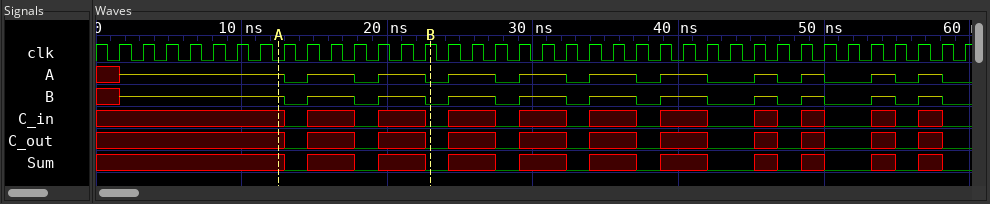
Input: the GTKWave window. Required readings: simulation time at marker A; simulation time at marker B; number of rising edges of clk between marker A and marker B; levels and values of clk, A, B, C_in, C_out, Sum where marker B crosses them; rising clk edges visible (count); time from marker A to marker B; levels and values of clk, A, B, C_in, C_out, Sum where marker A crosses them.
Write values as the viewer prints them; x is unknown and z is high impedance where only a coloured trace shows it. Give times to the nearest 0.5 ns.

12.5 ns
23 ns
7
clk=1, A=0, B=0, C_in=0, C_out=0, Sum=0
37
10.5 ns
clk=0, A=z, B=z, C_in=x, C_out=x, Sum=x
